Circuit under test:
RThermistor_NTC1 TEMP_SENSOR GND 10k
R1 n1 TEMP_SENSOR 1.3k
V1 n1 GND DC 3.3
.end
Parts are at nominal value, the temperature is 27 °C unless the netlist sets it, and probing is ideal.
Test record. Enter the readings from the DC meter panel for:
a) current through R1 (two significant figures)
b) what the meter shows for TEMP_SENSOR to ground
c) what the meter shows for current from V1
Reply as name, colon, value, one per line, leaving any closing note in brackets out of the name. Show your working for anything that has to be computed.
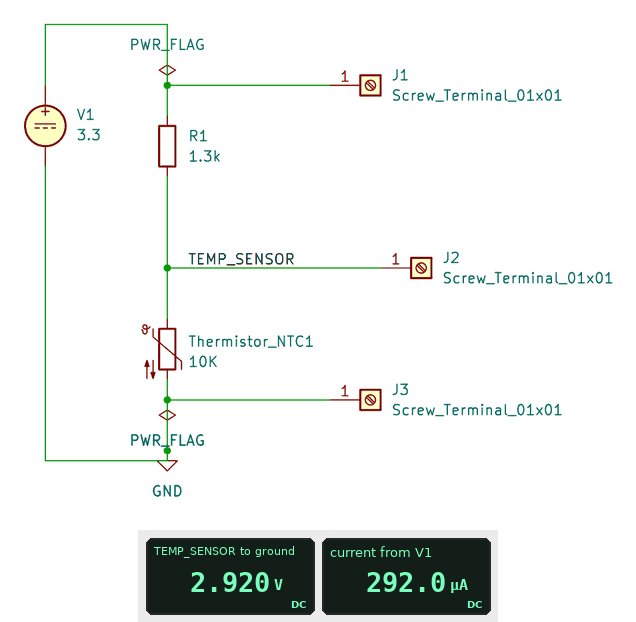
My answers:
current through R1: (3.3 V - 2.92 V) / 1.3 kΩ = 290 µA
what the meter shows for TEMP_SENSOR to ground: 2.920 V
what the meter shows for current from V1: 292.0 µA
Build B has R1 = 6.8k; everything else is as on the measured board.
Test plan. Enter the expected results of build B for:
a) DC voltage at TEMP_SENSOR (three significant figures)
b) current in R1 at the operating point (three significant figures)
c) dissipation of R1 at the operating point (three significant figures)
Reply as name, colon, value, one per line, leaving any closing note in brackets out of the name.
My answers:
DC voltage at TEMP_SENSOR: 1.96 V
current in R1 at the operating point: 196 µA
dissipation of R1 at the operating point: 262 µW
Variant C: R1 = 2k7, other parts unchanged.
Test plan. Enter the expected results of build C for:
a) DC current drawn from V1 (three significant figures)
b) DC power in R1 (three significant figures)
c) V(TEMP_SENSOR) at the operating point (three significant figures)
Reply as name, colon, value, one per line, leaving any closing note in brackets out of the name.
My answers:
DC current drawn from V1: 260 µA
DC power in R1: 182 µW
V(TEMP_SENSOR) at the operating point: 2.60 V
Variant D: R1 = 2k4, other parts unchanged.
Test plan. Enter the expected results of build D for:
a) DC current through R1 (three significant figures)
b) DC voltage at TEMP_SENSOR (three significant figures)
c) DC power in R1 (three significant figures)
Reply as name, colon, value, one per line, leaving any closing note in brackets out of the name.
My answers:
DC current through R1: 266 µA
DC voltage at TEMP_SENSOR: 2.66 V
DC power in R1: 170 µW
